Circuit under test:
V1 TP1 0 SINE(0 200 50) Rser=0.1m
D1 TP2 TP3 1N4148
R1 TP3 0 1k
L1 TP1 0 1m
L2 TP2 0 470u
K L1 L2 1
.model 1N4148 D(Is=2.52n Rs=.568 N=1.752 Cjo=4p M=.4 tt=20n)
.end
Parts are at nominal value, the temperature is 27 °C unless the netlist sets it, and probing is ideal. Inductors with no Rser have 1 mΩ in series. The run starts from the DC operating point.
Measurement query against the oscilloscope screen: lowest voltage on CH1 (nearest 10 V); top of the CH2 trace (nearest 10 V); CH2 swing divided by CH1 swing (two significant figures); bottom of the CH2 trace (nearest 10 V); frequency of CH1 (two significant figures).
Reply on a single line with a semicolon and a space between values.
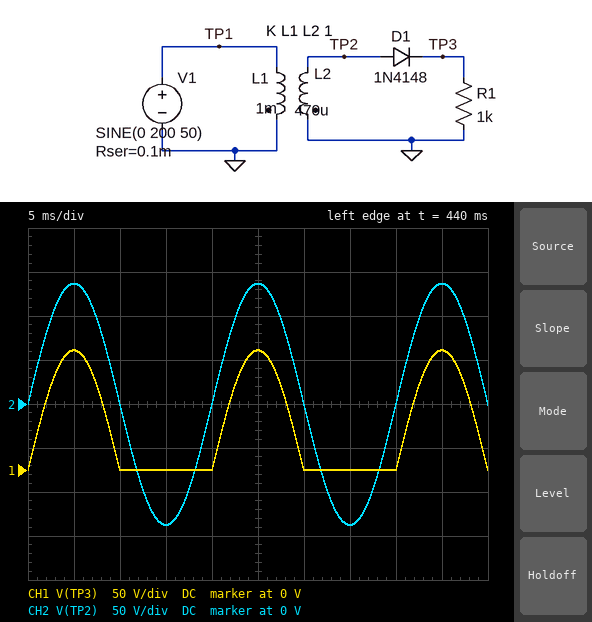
0 V; 140 V; 2.0; -140 V; 50 Hz
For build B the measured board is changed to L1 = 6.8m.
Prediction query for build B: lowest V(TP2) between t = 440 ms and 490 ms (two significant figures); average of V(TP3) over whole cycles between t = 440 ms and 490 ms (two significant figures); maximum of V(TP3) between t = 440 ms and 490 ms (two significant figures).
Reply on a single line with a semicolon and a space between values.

-53 V; 16 V; 52 V
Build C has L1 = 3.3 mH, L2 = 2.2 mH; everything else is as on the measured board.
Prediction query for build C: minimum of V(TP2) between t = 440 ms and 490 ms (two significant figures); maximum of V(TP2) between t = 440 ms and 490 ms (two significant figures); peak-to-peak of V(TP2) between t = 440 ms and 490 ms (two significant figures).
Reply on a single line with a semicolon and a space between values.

-160 V; 160 V; 330 V
